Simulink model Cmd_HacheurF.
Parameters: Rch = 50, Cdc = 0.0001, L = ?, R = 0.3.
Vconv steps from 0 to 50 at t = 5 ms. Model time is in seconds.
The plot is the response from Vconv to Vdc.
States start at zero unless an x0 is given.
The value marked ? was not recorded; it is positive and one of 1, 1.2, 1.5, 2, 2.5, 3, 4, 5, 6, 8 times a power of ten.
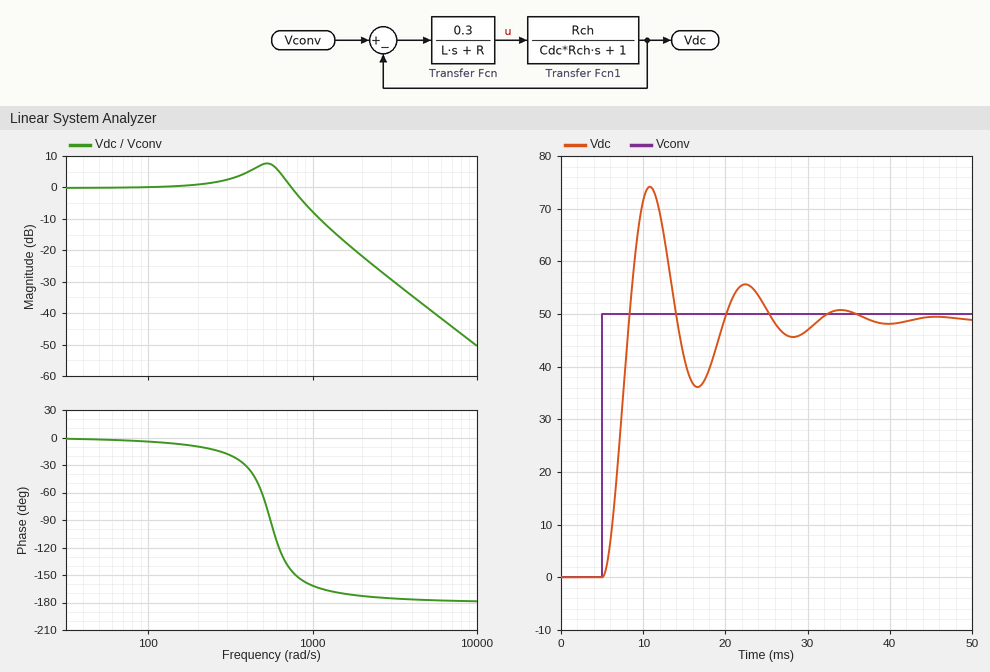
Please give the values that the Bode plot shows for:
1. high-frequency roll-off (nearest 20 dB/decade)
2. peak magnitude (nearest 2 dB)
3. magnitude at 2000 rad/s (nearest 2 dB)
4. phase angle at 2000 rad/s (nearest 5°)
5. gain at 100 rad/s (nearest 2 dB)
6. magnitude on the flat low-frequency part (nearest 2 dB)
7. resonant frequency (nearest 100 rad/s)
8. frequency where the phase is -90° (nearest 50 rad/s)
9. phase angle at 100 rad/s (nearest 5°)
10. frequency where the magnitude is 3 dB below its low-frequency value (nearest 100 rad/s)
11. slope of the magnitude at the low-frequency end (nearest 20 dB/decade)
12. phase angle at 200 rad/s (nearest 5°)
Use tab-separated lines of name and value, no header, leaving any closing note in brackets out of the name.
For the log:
high-frequency roll-off	-40 dB/decade
peak magnitude	8 dB
magnitude at 2000 rad/s	-22 dB
phase angle at 2000 rad/s	-175°
gain at 100 rad/s	0 dB
magnitude on the flat low-frequency part	0 dB
resonant frequency	500 rad/s
frequency where the phase is -90°	550 rad/s
phase angle at 100 rad/s	-5°
frequency where the magnitude is 3 dB below its low-frequency value	800 rad/s
slope of the magnitude at the low-frequency end	0 dB/decade
phase angle at 200 rad/s	-10°
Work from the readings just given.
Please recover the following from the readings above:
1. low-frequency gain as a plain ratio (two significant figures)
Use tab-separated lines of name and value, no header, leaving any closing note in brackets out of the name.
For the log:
low-frequency gain as a plain ratio	1.0
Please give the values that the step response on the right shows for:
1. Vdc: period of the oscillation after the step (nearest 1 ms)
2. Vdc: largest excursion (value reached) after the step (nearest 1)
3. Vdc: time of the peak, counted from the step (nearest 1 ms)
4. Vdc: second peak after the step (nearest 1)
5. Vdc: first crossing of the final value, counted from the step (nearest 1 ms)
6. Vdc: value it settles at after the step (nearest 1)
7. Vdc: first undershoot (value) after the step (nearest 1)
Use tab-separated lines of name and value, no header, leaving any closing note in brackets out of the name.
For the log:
Vdc: period of the oscillation after the step	12 ms
Vdc: largest excursion (value reached) after the step	74
Vdc: time of the peak, counted from the step	6 ms
Vdc: second peak after the step	56
Vdc: first crossing of the final value, counted from the step	3 ms
Vdc: value it settles at after the step	49
Vdc: first undershoot (value) after the step	36
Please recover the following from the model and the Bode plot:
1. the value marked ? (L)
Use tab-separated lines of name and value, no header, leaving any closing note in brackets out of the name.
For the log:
the value marked ?	0.01
